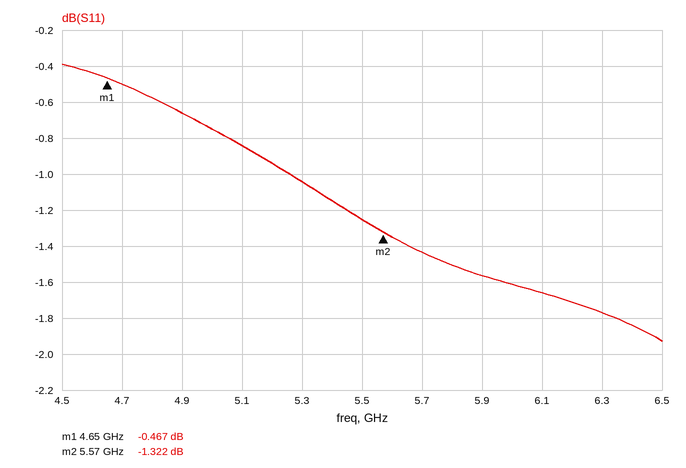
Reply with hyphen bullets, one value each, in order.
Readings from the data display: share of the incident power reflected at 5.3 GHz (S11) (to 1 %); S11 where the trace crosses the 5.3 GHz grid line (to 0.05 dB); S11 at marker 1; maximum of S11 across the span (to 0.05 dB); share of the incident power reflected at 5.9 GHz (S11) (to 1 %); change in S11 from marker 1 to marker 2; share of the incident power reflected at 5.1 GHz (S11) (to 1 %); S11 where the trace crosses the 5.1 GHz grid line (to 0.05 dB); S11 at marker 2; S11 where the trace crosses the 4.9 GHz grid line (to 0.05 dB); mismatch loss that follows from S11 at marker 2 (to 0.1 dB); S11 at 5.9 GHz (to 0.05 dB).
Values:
- 79 %
- -1.05 dB
- -0.467 dB
- -0.40 dB
- 70 %
- -0.855 dB
- 82 %
- -0.85 dB
- -1.322 dB
- -0.65 dB
- 5.8 dB
- -1.55 dB
